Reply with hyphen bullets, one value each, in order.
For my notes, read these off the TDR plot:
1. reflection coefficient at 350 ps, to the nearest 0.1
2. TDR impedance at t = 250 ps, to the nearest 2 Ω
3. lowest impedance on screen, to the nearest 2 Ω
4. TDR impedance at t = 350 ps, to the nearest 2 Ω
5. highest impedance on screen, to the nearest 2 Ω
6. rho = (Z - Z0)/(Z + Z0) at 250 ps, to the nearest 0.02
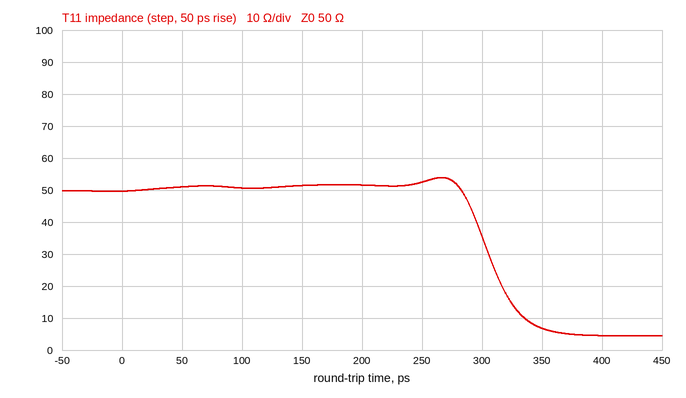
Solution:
- -0.8
- 52 Ω
- 4 Ω
- 6 Ω
- 54 Ω
- +0.02
